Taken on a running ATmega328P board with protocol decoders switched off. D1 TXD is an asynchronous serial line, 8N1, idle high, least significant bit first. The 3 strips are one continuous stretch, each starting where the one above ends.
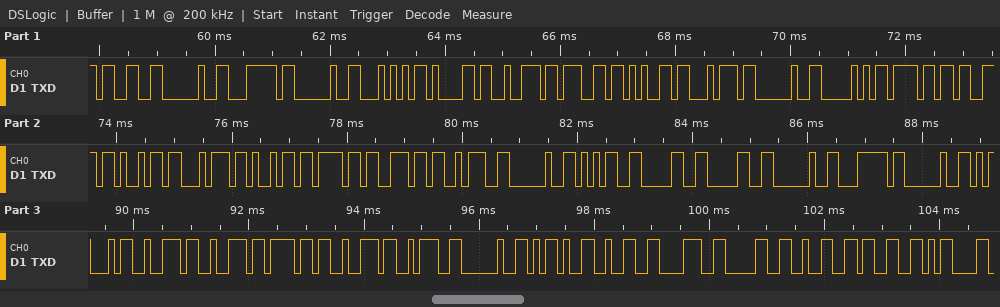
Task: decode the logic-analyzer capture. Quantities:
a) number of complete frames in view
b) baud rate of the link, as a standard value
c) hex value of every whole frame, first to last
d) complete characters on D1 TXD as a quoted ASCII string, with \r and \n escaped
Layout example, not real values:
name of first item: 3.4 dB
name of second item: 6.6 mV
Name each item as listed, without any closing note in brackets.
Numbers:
number of complete frames in view: 41
baud rate of the link, as a standard value: 9600 baud
hex value of every whole frame, first to last: 33 20 7C 20 54 61 72 67 65 74 20 50 6F 73 69 74 69 6F 6E 3A 20 35 30 30 20 7C 20 45 72 72 6F 72 3A 20 2D 32 38 30 32 33 0D
complete characters on D1 TXD as a quoted ASCII string, with \r and \n escaped: "3 | Target Position: 500 | Error: -28023\r"
